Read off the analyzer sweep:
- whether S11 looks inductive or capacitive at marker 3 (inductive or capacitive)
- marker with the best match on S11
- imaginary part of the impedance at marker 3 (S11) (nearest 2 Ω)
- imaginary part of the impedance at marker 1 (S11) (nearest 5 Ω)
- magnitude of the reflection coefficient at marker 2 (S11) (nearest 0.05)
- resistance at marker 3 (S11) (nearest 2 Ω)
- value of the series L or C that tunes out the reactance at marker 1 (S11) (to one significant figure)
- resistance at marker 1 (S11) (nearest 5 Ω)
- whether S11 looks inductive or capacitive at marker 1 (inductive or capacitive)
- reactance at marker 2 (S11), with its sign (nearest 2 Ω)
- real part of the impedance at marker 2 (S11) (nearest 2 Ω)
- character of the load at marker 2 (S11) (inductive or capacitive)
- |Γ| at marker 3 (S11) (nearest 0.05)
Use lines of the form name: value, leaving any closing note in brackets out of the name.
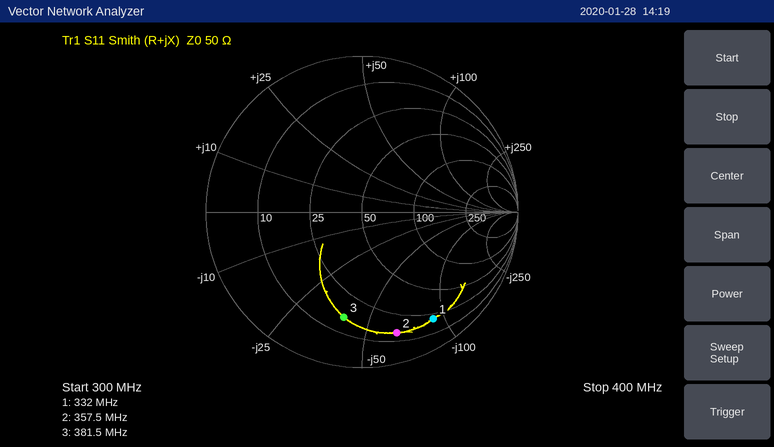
whether S11 looks inductive or capacitive at marker 3: capacitive
marker with the best match on S11: marker 3
imaginary part of the impedance at marker 3 (S11): -40 Ω
imaginary part of the impedance at marker 1 (S11): -90 Ω
magnitude of the reflection coefficient at marker 2 (S11): 0.80
resistance at marker 3 (S11): 16 Ω
value of the series L or C that tunes out the reactance at marker 1 (S11): 40 nH
resistance at marker 1 (S11): 20 Ω
whether S11 looks inductive or capacitive at marker 1: capacitive
reactance at marker 2 (S11), with its sign: -64 Ω
real part of the impedance at marker 2 (S11): 14 Ω
character of the load at marker 2 (S11): capacitive
|Γ| at marker 3 (S11): 0.70
